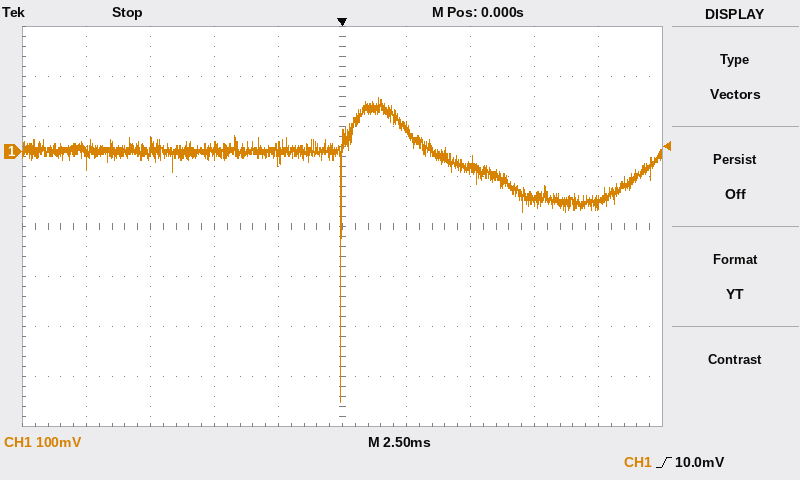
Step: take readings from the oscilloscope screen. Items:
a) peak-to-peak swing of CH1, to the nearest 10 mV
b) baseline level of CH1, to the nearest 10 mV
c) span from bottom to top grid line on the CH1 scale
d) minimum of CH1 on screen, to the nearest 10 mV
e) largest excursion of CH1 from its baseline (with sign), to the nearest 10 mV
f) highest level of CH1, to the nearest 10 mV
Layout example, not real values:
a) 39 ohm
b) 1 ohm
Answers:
a) 610 mV
b) 0 mV
c) 800 mV
d) -500 mV
e) -500 mV
f) 110 mV
